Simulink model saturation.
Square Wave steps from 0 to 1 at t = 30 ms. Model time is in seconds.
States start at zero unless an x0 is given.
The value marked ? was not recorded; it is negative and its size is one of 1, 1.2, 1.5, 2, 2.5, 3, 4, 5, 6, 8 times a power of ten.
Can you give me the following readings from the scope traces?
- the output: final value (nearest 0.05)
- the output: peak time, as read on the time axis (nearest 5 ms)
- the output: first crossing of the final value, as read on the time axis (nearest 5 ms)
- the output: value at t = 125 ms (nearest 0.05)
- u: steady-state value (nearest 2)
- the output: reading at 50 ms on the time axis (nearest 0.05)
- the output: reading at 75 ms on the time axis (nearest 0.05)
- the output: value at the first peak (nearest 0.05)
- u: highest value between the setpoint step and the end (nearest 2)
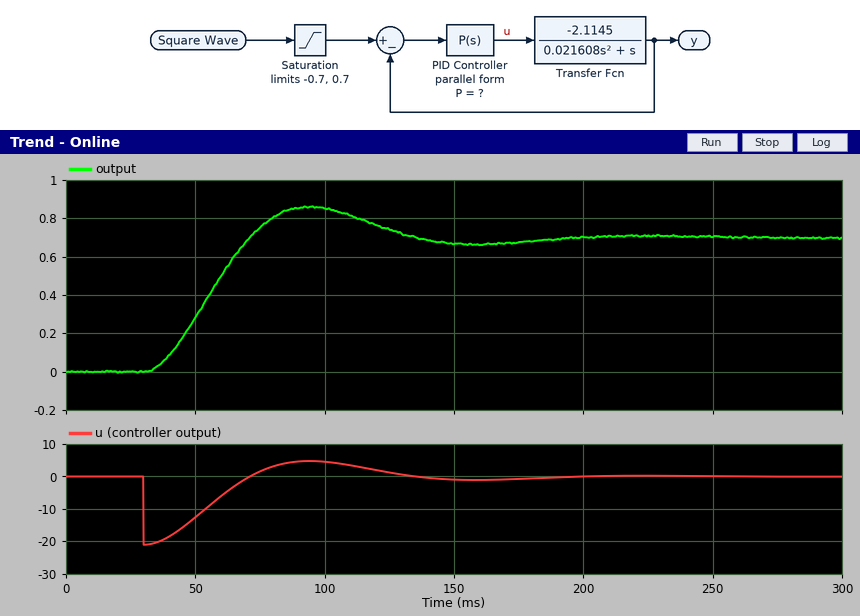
0.70
95 ms
70 ms
0.75
0
0.30
0.75
0.85
4
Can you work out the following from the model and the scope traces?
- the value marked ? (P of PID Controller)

-30
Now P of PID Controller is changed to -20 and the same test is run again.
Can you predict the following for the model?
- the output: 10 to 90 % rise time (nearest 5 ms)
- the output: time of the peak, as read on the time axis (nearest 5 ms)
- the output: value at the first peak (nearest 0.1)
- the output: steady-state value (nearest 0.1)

40 ms
115 ms
0.8
0.7
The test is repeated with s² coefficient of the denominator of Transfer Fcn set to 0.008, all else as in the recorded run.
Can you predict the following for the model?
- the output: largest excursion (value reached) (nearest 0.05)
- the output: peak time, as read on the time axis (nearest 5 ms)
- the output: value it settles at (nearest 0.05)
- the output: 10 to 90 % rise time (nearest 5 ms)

0.75
80 ms
0.70
25 ms
